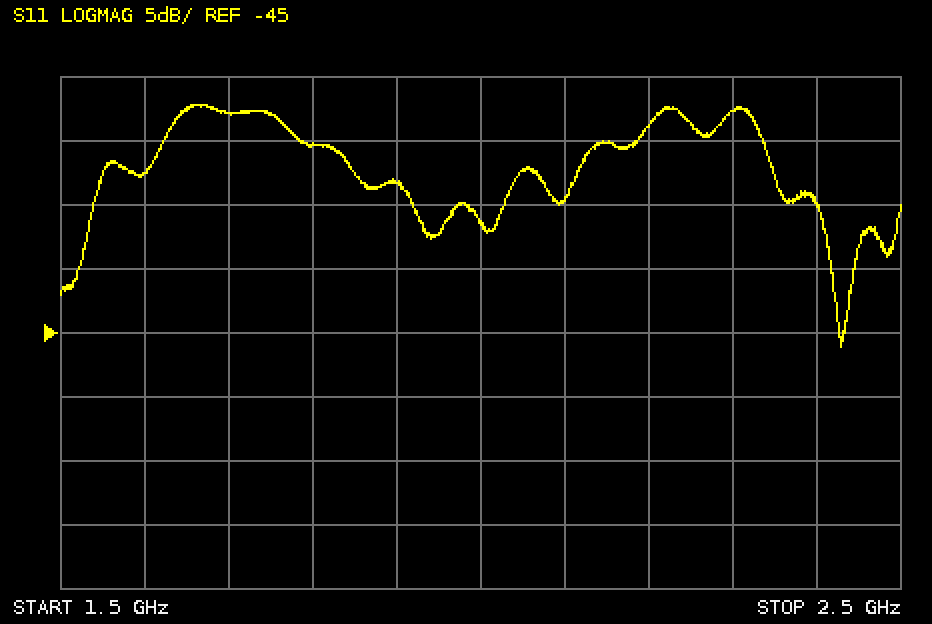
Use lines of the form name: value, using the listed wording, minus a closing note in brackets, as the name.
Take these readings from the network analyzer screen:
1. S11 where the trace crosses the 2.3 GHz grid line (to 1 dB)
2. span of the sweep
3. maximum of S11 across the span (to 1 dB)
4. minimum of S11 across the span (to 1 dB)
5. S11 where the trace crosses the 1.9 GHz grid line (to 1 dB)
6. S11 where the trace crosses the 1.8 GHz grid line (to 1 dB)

S11 where the trace crosses the 2.3 GHz grid line: -28 dB
span of the sweep: 1 GHz
maximum of S11 across the span: -27 dB
minimum of S11 across the span: -46 dB
S11 where the trace crosses the 1.9 GHz grid line: -33 dB
S11 where the trace crosses the 1.8 GHz grid line: -30 dB
